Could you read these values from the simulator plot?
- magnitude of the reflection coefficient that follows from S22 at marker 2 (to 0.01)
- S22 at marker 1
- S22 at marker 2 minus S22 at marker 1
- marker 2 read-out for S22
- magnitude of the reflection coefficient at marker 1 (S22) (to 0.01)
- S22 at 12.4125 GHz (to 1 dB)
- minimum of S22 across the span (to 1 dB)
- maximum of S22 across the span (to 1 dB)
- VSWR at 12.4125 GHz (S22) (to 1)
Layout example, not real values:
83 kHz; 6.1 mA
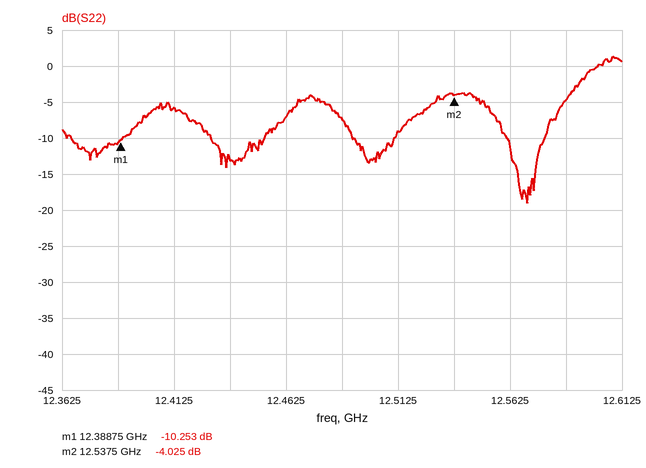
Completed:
0.63; -10.253 dB; 6.228 dB; -4.025 dB; 0.31; -6 dB; -19 dB; 1 dB; 3
